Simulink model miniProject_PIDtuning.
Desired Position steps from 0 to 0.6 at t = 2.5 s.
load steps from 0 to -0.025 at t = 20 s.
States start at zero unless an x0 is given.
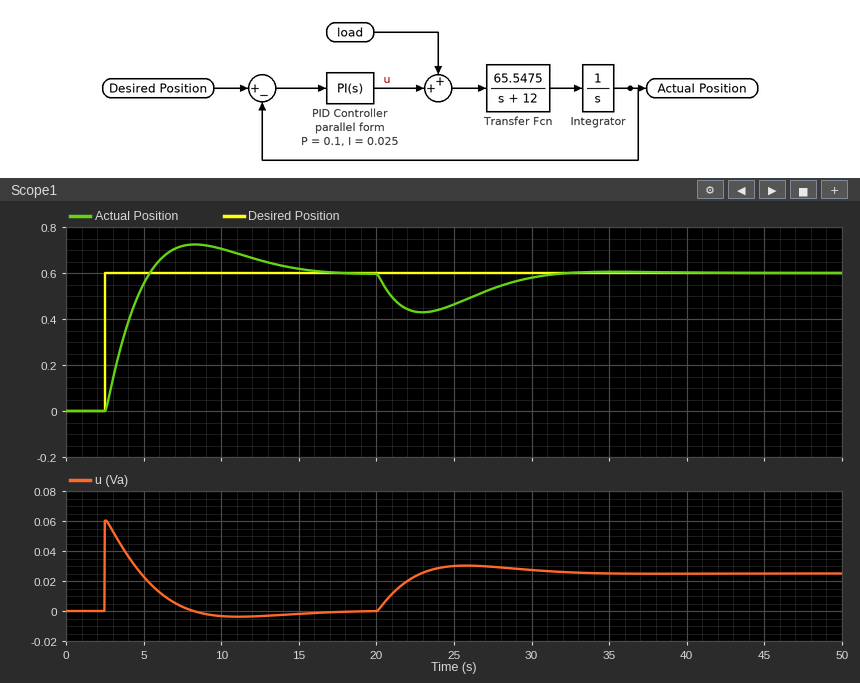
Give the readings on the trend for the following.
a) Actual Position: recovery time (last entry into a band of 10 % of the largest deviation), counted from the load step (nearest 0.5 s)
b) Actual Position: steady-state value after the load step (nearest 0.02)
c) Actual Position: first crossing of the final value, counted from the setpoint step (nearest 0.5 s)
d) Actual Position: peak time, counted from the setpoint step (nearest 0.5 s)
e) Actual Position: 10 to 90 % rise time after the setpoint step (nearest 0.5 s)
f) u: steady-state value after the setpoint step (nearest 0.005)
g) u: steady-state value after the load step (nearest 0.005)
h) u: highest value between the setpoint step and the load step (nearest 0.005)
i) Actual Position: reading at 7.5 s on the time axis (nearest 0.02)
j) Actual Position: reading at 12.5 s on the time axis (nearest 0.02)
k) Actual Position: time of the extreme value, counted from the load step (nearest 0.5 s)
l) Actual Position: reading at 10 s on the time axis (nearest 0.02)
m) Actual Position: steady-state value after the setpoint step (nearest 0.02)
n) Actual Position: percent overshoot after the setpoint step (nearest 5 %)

10.5 s
0.60
3.0 s
6.0 s
2.0 s
0.000
0.025
0.060
0.72
0.66
3.0 s
0.70
0.60
20 %
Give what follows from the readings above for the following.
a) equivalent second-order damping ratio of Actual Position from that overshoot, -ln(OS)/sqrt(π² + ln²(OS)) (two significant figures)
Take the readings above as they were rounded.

0.46
